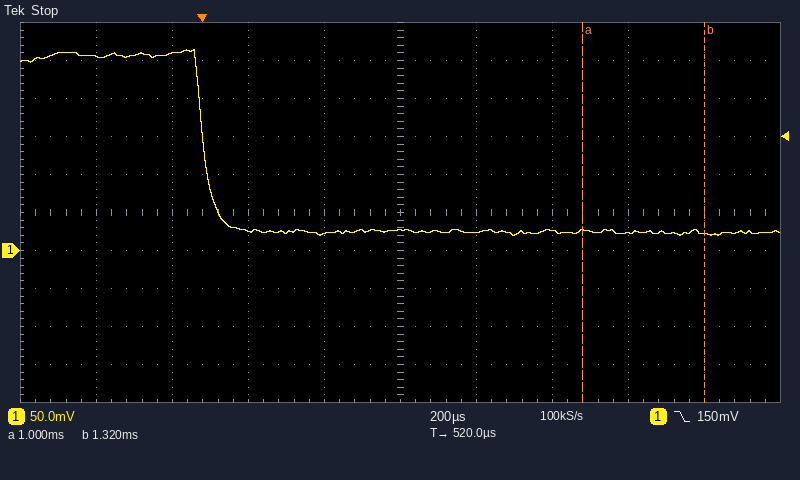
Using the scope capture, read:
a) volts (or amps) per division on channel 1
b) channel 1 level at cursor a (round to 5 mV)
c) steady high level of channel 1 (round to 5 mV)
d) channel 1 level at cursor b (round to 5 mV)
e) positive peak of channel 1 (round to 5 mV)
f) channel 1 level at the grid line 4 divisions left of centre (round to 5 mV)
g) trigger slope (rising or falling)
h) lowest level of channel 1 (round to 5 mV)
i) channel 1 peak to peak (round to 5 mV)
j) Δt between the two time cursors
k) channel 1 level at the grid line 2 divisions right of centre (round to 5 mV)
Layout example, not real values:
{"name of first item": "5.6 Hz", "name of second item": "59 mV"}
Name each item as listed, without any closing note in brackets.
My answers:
{"volts (or amps) per division on channel 1": "50 mV", "channel 1 level at cursor a": "25 mV", "steady high level of channel 1": "255 mV", "channel 1 level at cursor b": "20 mV", "positive peak of channel 1": "265 mV", "channel 1 level at the grid line 4 divisions left of centre": "255 mV", "trigger slope": "falling", "lowest level of channel 1": "20 mV", "channel 1 peak to peak": "245 mV", "Δt between the two time cursors": "320 µs", "channel 1 level at the grid line 2 divisions right of centre": "25 mV"}
